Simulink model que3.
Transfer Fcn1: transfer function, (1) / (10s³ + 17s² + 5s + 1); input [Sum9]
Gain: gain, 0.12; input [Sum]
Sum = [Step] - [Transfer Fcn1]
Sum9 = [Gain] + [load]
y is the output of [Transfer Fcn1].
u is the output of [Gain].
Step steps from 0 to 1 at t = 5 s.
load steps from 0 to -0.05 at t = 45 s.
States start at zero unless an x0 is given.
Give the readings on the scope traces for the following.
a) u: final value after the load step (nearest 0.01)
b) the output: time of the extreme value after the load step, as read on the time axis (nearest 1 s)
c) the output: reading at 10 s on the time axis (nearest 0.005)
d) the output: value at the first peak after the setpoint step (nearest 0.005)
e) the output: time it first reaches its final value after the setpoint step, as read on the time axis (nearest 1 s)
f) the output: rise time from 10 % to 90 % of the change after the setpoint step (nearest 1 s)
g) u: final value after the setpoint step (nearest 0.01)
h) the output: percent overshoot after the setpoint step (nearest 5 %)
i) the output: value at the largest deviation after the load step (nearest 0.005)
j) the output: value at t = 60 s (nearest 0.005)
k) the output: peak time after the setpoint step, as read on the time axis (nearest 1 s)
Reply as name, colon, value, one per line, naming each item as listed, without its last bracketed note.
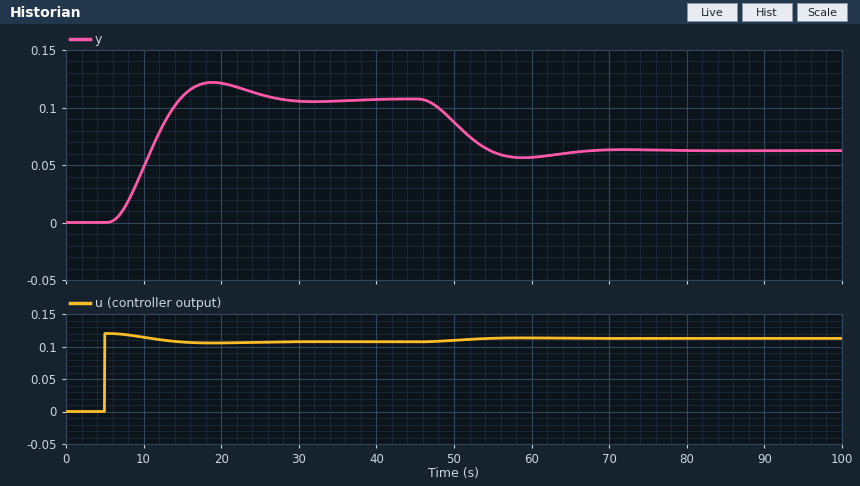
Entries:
u: final value after the load step: 0.11
the output: time of the extreme value after the load step, as read on the time axis: 59 s
the output: reading at 10 s on the time axis: 0.050
the output: value at the first peak after the setpoint step: 0.120
the output: time it first reaches its final value after the setpoint step, as read on the time axis: 15 s
the output: rise time from 10 % to 90 % of the change after the setpoint step: 6 s
u: final value after the setpoint step: 0.11
the output: percent overshoot after the setpoint step: 15 %
the output: value at the largest deviation after the load step: 0.055
the output: value at t = 60 s: 0.055
the output: peak time after the setpoint step, as read on the time axis: 19 s
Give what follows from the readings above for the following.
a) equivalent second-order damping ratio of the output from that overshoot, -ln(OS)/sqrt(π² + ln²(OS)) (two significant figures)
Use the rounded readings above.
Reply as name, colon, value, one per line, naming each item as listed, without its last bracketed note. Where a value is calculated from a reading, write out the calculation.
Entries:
equivalent second-order damping ratio of the output from that overshoot, -ln(OS)/sqrt(π² + ln²(OS)): ln(0.15) = -1.897; 1.897 / sqrt(9.870 + 3.599) = 0.52
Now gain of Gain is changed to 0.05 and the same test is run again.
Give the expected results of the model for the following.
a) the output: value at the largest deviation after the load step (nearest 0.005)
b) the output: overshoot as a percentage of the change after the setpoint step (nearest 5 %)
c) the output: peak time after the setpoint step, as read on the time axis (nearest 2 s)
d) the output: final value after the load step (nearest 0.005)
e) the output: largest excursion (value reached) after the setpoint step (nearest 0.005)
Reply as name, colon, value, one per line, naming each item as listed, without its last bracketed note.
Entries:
the output: value at the largest deviation after the load step: -0.005
the output: overshoot as a percentage of the change after the setpoint step: 10 %
the output: peak time after the setpoint step, as read on the time axis: 20 s
the output: final value after the load step: 0.000
the output: largest excursion (value reached) after the setpoint step: 0.055
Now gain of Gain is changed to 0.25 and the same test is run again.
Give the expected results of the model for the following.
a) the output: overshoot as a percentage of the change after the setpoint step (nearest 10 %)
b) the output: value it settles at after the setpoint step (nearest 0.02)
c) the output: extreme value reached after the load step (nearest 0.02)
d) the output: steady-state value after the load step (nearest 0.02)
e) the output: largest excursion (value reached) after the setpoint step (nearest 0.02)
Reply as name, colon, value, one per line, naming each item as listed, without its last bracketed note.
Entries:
the output: overshoot as a percentage of the change after the setpoint step: 20 %
the output: value it settles at after the setpoint step: 0.20
the output: extreme value reached after the load step: 0.16
the output: steady-state value after the load step: 0.16
the output: largest excursion (value reached) after the setpoint step: 0.24
